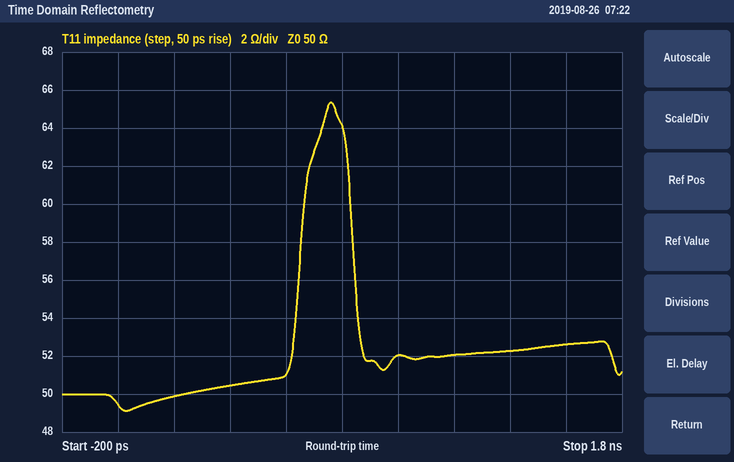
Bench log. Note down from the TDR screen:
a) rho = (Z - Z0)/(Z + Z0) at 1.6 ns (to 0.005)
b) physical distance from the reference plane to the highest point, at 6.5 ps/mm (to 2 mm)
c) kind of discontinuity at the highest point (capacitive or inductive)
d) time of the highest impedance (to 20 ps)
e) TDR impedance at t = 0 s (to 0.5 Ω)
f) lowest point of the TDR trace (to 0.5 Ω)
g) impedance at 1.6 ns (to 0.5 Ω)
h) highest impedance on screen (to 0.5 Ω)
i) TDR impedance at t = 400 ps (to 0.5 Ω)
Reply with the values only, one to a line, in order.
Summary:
+0.025
58 mm
inductive
760 ps
49.5 Ω
49.0 Ω
52.5 Ω
65.5 Ω
50.5 Ω
